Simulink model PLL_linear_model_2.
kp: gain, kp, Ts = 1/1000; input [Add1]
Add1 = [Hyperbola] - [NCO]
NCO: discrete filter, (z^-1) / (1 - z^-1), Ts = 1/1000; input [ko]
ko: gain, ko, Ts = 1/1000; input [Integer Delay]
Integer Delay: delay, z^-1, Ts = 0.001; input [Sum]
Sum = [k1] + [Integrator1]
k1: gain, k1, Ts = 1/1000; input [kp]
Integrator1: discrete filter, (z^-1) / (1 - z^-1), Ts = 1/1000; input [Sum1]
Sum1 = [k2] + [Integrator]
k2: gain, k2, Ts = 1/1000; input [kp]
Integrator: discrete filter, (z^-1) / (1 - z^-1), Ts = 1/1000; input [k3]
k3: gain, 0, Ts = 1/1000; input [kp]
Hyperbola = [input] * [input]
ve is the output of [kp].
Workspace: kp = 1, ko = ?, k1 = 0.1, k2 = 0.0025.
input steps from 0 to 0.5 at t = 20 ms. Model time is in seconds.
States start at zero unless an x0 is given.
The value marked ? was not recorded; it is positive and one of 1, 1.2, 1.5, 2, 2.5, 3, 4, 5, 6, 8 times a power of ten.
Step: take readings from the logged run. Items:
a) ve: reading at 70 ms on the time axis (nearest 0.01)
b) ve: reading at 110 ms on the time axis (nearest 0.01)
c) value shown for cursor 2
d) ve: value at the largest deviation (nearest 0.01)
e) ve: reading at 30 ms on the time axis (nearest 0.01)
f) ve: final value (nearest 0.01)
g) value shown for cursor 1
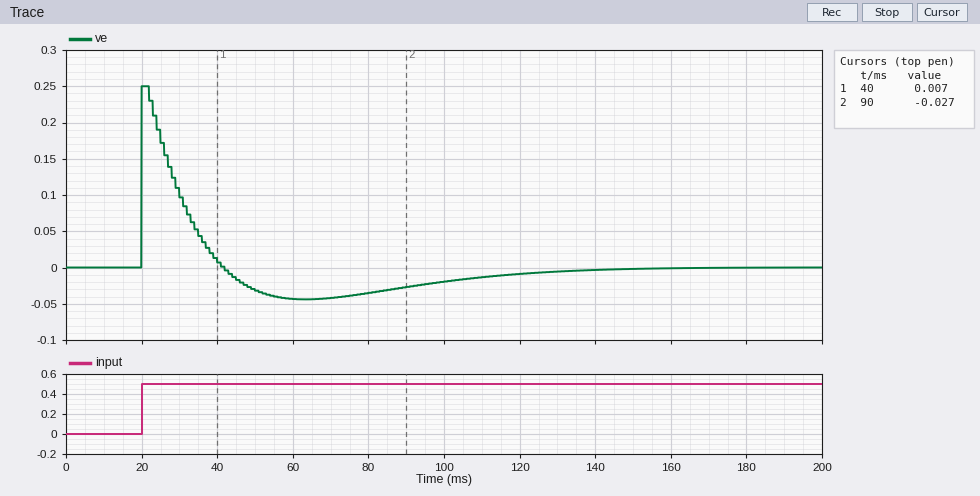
-0.04
-0.01
-0.027
0.25
0.10
0.00
0.007
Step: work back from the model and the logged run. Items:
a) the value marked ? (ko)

0.8
